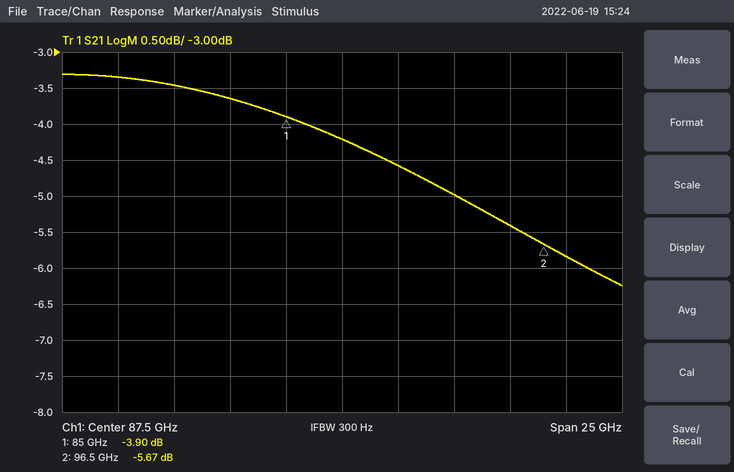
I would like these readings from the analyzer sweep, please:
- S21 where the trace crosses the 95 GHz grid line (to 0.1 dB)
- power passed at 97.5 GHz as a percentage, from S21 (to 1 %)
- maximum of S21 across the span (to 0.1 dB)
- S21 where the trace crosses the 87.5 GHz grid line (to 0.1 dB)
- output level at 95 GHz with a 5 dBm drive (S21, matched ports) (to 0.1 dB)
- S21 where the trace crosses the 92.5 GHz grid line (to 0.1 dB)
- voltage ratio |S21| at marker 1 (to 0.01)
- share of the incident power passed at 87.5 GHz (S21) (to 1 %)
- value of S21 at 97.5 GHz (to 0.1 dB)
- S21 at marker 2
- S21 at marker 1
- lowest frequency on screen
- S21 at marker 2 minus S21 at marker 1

-5.4 dB
26 %
-3.3 dB
-4.2 dB
-0.4 dBm
-5.0 dB
0.64
38 %
-5.8 dB
-5.67 dB
-3.90 dB
75 GHz
-1.77 dB
